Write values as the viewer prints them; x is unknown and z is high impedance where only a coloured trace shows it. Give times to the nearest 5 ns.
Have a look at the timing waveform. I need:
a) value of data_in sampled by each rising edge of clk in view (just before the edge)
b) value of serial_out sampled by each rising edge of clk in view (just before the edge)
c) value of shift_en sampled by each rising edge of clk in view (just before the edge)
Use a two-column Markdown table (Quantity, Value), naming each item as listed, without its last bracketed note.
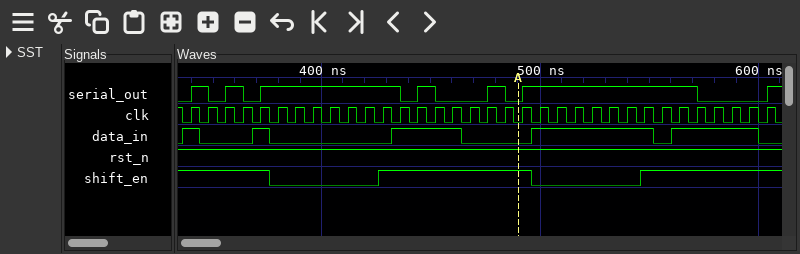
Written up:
| Quantity | Value |
|---|---|
| value of data_in sampled by each rising edge of clk in view | 1 0 0 0 1 0 0 0 0 0 0 0 1 1 1 1 0 0 0 0 1 1 1 1 1 1 1 0 1 1 1 1 1 0 |
| value of serial_out sampled by each rising edge of clk in view | 0 1 0 1 0 1 1 1 1 1 1 1 1 0 1 0 0 0 1 0 1 1 1 1 1 1 1 1 1 1 0 0 0 0 |
| value of shift_en sampled by each rising edge of clk in view | 1 1 1 1 1 0 0 0 0 0 0 1 1 1 1 1 1 1 1 1 0 0 0 0 0 0 1 1 1 1 1 1 1 1 |
